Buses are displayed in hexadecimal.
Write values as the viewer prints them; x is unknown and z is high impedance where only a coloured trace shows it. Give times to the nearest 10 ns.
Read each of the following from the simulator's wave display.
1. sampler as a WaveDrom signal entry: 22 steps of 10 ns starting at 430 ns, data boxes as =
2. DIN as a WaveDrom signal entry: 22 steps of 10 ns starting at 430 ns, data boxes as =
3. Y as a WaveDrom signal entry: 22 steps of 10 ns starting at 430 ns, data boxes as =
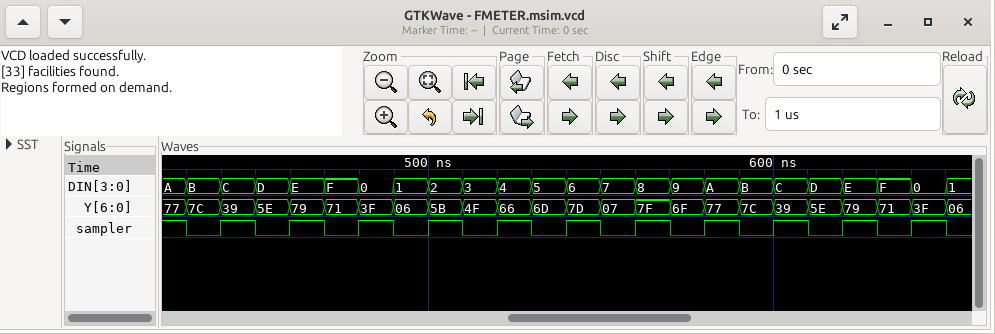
{name: 'sampler', wave: '0101010101010101010101'}
{name: 'DIN', wave: '======================', data: 'B C D E F 0 1 2 3 4 5 6 7 8 9 A B C D E F 0'}
{name: 'Y', wave: '======================', data: '7C 39 5E 79 71 3F 06 5B 4F 66 6D 7D 07 7F 6F 77 7C 39 5E 79 71 3F'}
